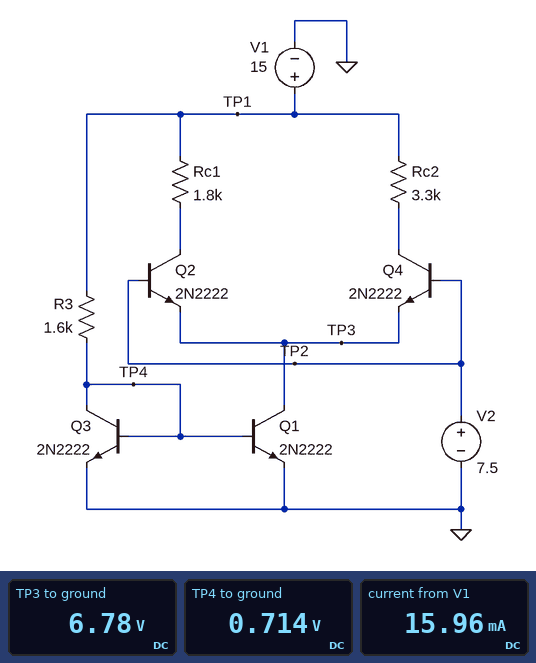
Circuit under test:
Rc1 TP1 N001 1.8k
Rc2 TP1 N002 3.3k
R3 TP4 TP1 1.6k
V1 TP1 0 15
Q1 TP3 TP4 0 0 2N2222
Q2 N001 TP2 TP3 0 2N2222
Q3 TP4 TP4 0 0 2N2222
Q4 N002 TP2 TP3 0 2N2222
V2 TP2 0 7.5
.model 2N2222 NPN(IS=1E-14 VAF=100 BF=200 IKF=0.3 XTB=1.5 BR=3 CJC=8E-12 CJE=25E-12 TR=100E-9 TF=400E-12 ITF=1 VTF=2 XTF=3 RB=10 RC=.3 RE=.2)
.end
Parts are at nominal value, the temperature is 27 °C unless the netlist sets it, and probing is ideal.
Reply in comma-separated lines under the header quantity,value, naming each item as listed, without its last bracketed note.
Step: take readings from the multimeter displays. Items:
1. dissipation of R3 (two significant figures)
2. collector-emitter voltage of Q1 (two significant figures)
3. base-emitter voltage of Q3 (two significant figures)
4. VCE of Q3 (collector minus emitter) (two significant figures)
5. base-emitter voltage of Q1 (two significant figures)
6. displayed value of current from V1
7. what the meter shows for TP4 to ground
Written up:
quantity,value
dissipation of R3,130 mW
collector-emitter voltage of Q1,6.8 V
base-emitter voltage of Q3,710 mV
VCE of Q3 (collector minus emitter),710 mV
base-emitter voltage of Q1,710 mV
displayed value of current from V1,15.96 mA
what the meter shows for TP4 to ground,0.714 V
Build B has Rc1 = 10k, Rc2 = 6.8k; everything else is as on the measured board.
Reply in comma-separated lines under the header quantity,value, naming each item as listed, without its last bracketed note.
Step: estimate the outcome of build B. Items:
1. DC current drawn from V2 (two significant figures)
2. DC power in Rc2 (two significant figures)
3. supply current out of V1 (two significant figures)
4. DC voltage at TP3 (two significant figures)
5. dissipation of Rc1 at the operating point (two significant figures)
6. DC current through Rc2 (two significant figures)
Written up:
quantity,value
DC current drawn from V2,7.3 mA
DC power in Rc2,10 mW
supply current out of V1,11 mA
DC voltage at TP3,6.7 V
dissipation of Rc1 at the operating point,6.8 mW
DC current through Rc2,1.2 mA
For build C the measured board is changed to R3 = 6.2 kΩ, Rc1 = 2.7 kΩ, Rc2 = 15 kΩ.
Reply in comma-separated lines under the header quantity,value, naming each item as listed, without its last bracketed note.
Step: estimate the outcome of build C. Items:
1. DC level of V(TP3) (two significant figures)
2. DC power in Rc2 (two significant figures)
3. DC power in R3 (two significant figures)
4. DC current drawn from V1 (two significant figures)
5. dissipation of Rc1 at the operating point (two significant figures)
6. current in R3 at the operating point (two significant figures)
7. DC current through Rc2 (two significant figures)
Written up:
quantity,value
DC level of V(TP3),6.8 V
DC power in Rc2,4.4 mW
DC power in R3,33 mW
DC current drawn from V1,4.5 mA
dissipation of Rc1 at the operating point,7.2 mW
current in R3 at the operating point,2.3 mA
DC current through Rc2,540 µA
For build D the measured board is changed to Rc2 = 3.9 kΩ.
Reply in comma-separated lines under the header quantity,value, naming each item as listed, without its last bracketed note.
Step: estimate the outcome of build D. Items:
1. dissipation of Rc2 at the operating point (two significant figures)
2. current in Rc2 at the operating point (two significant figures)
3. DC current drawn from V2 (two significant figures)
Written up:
quantity,value
dissipation of Rc2 at the operating point,17 mW
current in Rc2 at the operating point,2.1 mA
DC current drawn from V2,2.7 mA
